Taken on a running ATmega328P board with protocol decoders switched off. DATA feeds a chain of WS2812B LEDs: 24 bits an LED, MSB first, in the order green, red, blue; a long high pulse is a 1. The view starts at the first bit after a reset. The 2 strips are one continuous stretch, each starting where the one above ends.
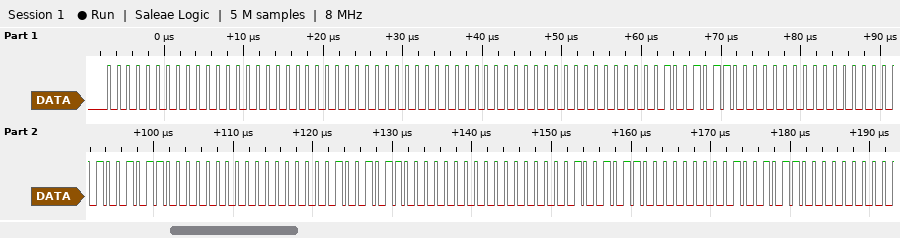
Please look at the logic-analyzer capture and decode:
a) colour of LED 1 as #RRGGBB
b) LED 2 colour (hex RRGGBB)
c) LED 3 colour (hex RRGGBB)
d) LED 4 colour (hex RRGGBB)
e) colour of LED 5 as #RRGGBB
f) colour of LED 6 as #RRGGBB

#000000
#000000
#960000
#960000
#960000
#960000
